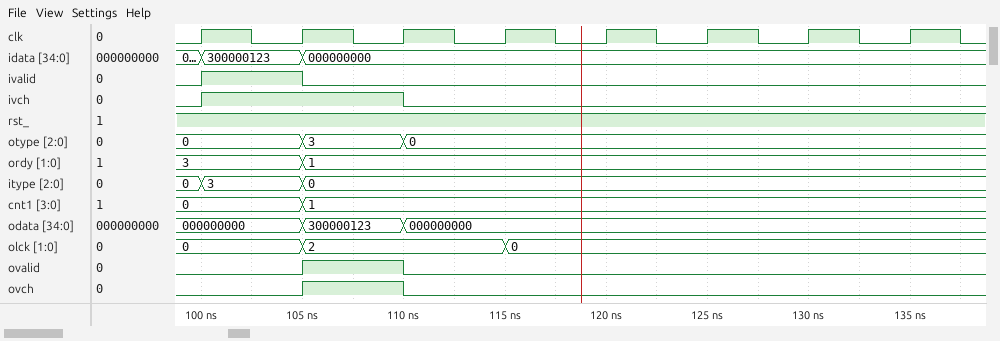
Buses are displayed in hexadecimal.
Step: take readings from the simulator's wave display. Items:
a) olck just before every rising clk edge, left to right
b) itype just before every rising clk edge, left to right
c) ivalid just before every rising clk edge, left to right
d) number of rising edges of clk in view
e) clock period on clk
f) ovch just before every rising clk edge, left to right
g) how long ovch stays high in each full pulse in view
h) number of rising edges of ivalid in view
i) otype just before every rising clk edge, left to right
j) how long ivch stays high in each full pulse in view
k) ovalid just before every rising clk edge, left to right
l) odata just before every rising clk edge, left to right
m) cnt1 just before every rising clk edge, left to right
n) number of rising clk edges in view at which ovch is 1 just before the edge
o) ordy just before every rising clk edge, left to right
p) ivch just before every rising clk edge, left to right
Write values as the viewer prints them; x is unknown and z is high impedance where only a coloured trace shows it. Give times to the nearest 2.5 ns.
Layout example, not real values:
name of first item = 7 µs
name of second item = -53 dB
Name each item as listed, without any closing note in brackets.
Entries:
olck just before every rising clk edge, left to right = 0, 0, 2, 2, 0, 0, 0, 0
itype just before every rising clk edge, left to right = 0, 3, 0, 0, 0, 0, 0, 0
ivalid just before every rising clk edge, left to right = 0 1 0 0 0 0 0 0
number of rising edges of clk in view = 8
clock period on clk = 5 ns
ovch just before every rising clk edge, left to right = 0 0 1 0 0 0 0 0
how long ovch stays high in each full pulse in view = 5 ns
number of rising edges of ivalid in view = 1
otype just before every rising clk edge, left to right = 0, 0, 3, 0, 0, 0, 0, 0
how long ivch stays high in each full pulse in view = 10 ns
ovalid just before every rising clk edge, left to right = 0 0 1 0 0 0 0 0
odata just before every rising clk edge, left to right = 000000000, 000000000, 300000123, 000000000, 000000000, 000000000, 000000000, 000000000
cnt1 just before every rising clk edge, left to right = 0, 0, 1, 1, 1, 1, 1, 1
number of rising clk edges in view at which ovch is 1 just before the edge = 1
ordy just before every rising clk edge, left to right = 3, 3, 1, 1, 1, 1, 1, 1
ivch just before every rising clk edge, left to right = 0 1 1 0 0 0 0 0
